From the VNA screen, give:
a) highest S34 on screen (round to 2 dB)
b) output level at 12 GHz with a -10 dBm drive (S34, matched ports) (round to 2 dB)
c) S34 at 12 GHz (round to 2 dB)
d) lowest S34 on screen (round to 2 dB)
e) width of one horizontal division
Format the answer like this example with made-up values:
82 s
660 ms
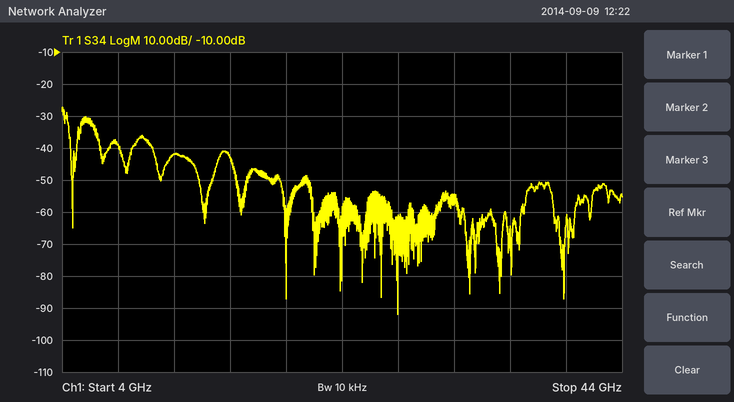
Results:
-28 dB
-52 dBm
-42 dB
-92 dB
4 GHz
